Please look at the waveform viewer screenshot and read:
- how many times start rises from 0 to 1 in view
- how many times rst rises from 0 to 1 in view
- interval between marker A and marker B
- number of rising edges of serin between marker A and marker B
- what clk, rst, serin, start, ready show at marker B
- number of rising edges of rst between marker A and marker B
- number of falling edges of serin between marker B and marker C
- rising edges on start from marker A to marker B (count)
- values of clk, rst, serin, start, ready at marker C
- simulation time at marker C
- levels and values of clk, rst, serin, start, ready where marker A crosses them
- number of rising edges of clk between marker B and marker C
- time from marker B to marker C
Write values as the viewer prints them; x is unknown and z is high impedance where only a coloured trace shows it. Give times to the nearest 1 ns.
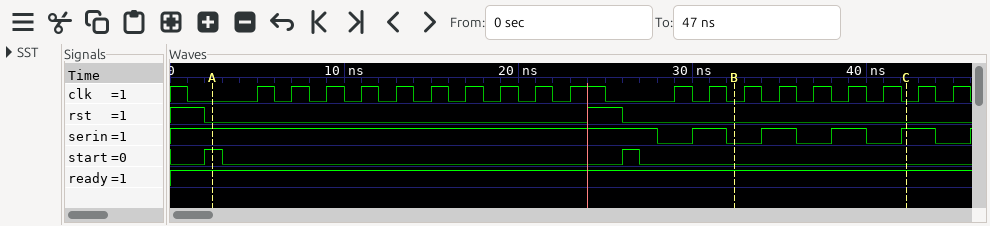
2
1
30 ns
1
clk=0, rst=0, serin=0, start=0, ready=1
1
2
1
clk=0, rst=0, serin=1, start=0, ready=1
42 ns
clk=0, rst=0, serin=1, start=1, ready=1
5
10 ns
